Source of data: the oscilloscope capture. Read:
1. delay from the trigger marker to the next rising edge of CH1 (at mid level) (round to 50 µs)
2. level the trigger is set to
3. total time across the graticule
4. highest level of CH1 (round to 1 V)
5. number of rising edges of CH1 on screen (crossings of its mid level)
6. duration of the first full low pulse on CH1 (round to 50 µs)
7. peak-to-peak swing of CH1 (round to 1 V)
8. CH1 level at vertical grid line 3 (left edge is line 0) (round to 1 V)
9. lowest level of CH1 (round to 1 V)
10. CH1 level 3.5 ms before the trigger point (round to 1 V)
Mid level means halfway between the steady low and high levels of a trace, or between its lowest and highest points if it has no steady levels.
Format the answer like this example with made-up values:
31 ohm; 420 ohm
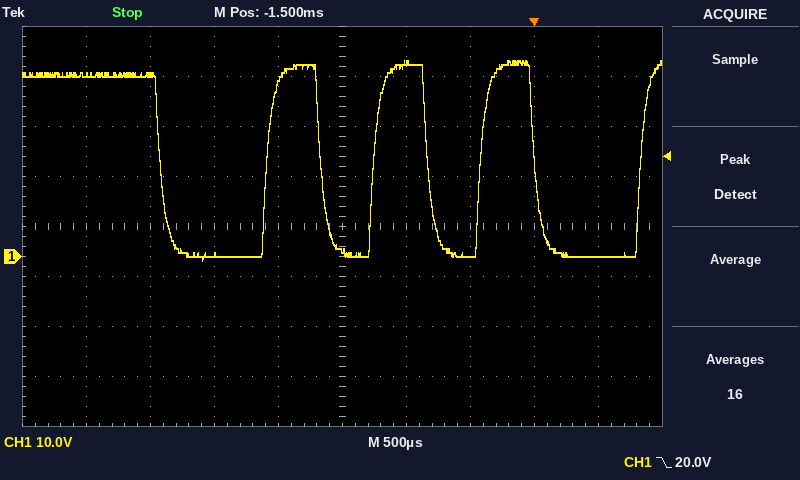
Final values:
850 µs; 20.0 V; 5 ms; 39 V; 4; 850 µs; 40 V; 0 V; -1 V; 36 V
